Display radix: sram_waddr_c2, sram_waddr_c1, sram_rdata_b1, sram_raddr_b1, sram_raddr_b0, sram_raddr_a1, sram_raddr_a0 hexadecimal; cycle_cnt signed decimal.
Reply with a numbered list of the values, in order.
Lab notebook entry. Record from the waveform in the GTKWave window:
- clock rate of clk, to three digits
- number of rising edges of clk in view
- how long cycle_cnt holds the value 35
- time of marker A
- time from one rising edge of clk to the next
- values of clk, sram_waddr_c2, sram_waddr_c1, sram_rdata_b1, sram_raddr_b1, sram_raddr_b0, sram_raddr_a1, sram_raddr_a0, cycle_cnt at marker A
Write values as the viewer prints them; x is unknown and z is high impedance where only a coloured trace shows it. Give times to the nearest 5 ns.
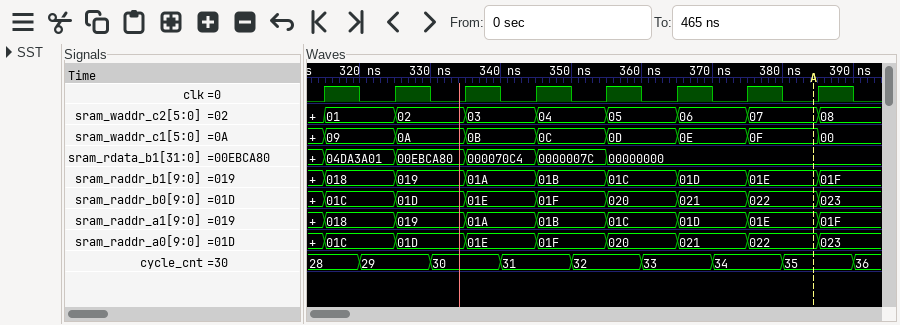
1. 100 MHz
2. 8
3. 10 ns
4. 385 ns
5. 10 ns
6. clk=0, sram_waddr_c2=07, sram_waddr_c1=0F, sram_rdata_b1=00000000, sram_raddr_b1=01E, sram_raddr_b0=022, sram_raddr_a1=01E, sram_raddr_a0=022, cycle_cnt=35
